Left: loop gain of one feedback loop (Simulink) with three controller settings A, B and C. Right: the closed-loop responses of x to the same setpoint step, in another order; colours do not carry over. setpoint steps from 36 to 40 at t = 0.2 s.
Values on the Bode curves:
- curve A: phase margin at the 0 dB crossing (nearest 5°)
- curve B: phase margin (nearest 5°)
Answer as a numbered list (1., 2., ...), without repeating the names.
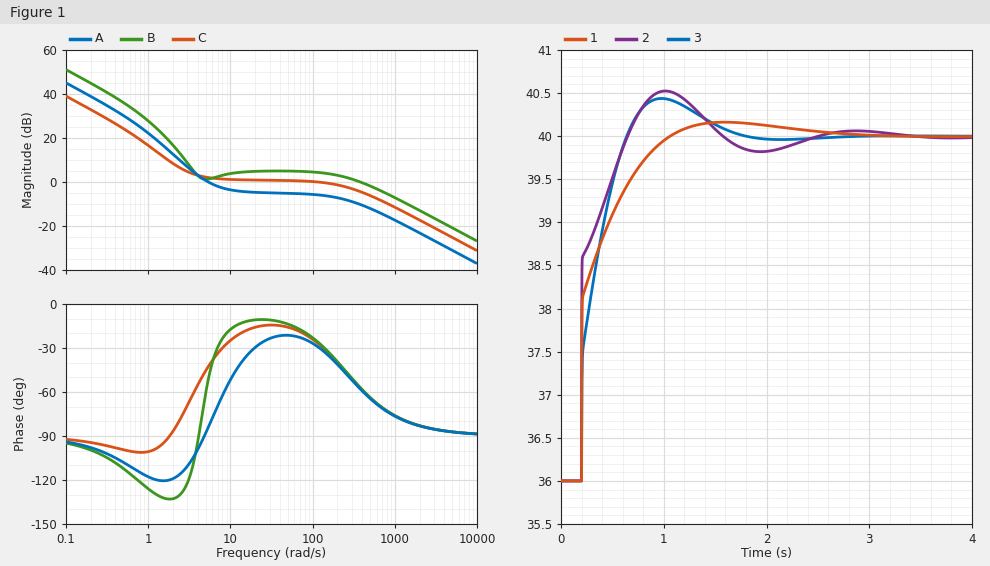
1. 95°
2. 125°
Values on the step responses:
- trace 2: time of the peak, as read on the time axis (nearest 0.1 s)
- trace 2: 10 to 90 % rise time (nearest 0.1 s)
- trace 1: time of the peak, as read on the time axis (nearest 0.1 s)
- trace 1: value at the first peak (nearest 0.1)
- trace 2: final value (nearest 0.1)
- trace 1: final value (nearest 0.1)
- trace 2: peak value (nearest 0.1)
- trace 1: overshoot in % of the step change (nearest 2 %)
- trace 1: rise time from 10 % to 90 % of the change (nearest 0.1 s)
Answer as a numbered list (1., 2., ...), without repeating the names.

1. 1.0 s
2. 0.3 s
3. 1.6 s
4. 40.2
5. 40.0
6. 40.0
7. 40.5
8. 4 %
9. 0.5 s
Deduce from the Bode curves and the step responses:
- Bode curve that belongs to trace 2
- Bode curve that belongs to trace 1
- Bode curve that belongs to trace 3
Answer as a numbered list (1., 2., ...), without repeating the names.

1. B
2. C
3. A
